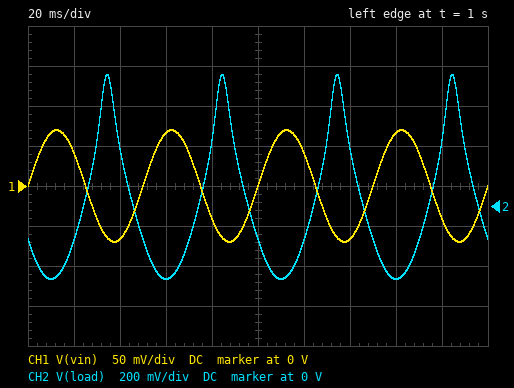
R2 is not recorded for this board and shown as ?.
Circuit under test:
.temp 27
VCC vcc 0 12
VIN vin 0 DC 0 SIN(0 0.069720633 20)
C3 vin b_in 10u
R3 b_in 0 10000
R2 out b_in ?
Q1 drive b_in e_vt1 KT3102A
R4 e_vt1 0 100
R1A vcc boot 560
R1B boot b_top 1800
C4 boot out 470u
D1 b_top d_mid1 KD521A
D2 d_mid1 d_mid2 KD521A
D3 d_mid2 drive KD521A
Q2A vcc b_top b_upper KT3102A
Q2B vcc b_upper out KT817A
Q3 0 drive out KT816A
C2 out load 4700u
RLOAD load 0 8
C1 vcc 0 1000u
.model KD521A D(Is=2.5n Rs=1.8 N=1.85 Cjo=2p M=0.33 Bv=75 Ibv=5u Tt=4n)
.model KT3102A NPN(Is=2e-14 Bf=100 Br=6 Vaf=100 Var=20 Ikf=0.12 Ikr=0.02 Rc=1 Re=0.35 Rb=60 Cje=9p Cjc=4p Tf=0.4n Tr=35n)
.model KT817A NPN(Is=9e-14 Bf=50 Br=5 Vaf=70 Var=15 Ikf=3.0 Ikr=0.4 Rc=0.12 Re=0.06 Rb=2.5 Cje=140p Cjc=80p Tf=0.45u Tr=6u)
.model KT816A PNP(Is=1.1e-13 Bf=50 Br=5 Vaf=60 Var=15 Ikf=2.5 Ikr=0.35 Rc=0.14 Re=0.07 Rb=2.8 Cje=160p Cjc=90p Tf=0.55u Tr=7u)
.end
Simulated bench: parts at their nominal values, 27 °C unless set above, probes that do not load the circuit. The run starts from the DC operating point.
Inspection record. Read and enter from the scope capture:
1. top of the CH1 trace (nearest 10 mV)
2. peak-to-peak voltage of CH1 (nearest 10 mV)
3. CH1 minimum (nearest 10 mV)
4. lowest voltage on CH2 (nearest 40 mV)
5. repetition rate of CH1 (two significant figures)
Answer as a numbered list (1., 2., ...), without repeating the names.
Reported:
1. 70 mV
2. 140 mV
3. -70 mV
4. -360 mV
5. 20 Hz
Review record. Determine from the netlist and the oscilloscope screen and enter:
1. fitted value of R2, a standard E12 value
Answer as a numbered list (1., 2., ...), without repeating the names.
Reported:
1. 39 kΩ
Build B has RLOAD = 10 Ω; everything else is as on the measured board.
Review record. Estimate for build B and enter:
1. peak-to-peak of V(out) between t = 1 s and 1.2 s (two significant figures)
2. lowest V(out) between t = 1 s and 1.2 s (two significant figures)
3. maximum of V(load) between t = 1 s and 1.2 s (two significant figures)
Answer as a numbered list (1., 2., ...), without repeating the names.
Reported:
1. 1.2 V
2. 5.2 V
3. 790 mV
